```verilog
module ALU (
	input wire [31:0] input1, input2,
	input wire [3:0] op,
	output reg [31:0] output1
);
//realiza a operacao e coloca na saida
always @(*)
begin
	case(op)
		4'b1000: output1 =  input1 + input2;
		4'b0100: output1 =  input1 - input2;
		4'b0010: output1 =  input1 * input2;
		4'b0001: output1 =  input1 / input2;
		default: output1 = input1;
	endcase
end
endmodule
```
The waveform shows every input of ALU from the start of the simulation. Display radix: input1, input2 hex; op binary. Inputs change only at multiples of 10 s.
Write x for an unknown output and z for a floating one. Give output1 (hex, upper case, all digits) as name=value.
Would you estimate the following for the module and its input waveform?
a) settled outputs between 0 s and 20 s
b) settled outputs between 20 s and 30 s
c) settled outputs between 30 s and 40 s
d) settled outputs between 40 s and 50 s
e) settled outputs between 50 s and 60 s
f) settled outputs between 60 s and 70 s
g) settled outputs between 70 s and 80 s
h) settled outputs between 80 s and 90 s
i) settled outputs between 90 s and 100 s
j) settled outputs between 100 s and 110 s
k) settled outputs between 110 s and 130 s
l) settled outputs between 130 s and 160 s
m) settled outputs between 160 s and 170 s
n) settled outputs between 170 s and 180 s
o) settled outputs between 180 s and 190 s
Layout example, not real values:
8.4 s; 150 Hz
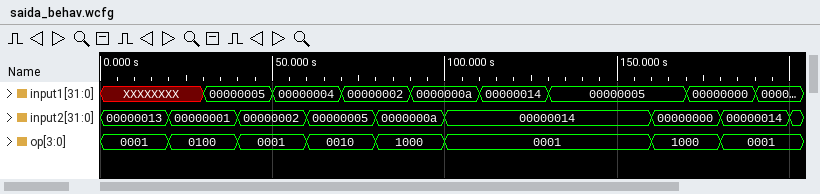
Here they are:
output1=x; output1=x; output1=00000004; output1=00000002; output1=00000002; output1=00000014; output1=0000000A; output1=0000000C; output1=00000014; output1=00000000; output1=00000001; output1=00000000; output1=00000005; output1=00000000; output1=00000000
